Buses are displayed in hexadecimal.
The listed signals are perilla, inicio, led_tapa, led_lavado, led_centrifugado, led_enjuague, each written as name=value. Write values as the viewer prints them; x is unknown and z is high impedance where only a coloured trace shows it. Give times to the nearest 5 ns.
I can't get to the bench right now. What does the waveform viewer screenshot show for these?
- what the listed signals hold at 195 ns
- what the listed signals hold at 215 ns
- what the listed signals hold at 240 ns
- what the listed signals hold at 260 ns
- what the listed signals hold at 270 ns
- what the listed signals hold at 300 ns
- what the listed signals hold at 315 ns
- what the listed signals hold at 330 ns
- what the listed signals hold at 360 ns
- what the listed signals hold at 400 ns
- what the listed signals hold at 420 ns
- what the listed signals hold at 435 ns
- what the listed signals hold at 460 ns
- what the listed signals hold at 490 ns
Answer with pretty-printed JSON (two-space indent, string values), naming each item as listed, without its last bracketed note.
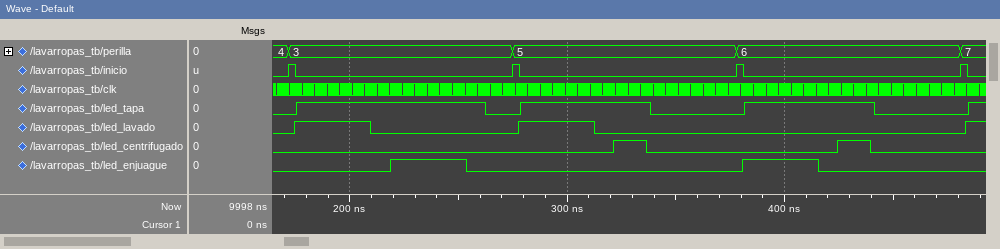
{
  "what the listed signals hold at 195 ns": "perilla=3, inicio=0, led_tapa=1, led_lavado=1, led_centrifugado=0, led_enjuague=0",
  "what the listed signals hold at 215 ns": "perilla=3, inicio=0, led_tapa=1, led_lavado=0, led_centrifugado=0, led_enjuague=0",
  "what the listed signals hold at 240 ns": "perilla=3, inicio=0, led_tapa=1, led_lavado=0, led_centrifugado=0, led_enjuague=1",
  "what the listed signals hold at 260 ns": "perilla=3, inicio=0, led_tapa=1, led_lavado=0, led_centrifugado=0, led_enjuague=0",
  "what the listed signals hold at 270 ns": "perilla=3, inicio=0, led_tapa=0, led_lavado=0, led_centrifugado=0, led_enjuague=0",
  "what the listed signals hold at 300 ns": "perilla=5, inicio=0, led_tapa=1, led_lavado=1, led_centrifugado=0, led_enjuague=0",
  "what the listed signals hold at 315 ns": "perilla=5, inicio=0, led_tapa=1, led_lavado=0, led_centrifugado=0, led_enjuague=0",
  "what the listed signals hold at 330 ns": "perilla=5, inicio=0, led_tapa=1, led_lavado=0, led_centrifugado=1, led_enjuague=0",
  "what the listed signals hold at 360 ns": "perilla=5, inicio=0, led_tapa=0, led_lavado=0, led_centrifugado=0, led_enjuague=0",
  "what the listed signals hold at 400 ns": "perilla=6, inicio=0, led_tapa=1, led_lavado=0, led_centrifugado=0, led_enjuague=1",
  "what the listed signals hold at 420 ns": "perilla=6, inicio=0, led_tapa=1, led_lavado=0, led_centrifugado=0, led_enjuague=0",
  "what the listed signals hold at 435 ns": "perilla=6, inicio=0, led_tapa=1, led_lavado=0, led_centrifugado=1, led_enjuague=0",
  "what the listed signals hold at 460 ns": "perilla=6, inicio=0, led_tapa=0, led_lavado=0, led_centrifugado=0, led_enjuague=0",
  "what the listed signals hold at 490 ns": "perilla=7, inicio=0, led_tapa=1, led_lavado=1, led_centrifugado=0, led_enjuague=0"
}
